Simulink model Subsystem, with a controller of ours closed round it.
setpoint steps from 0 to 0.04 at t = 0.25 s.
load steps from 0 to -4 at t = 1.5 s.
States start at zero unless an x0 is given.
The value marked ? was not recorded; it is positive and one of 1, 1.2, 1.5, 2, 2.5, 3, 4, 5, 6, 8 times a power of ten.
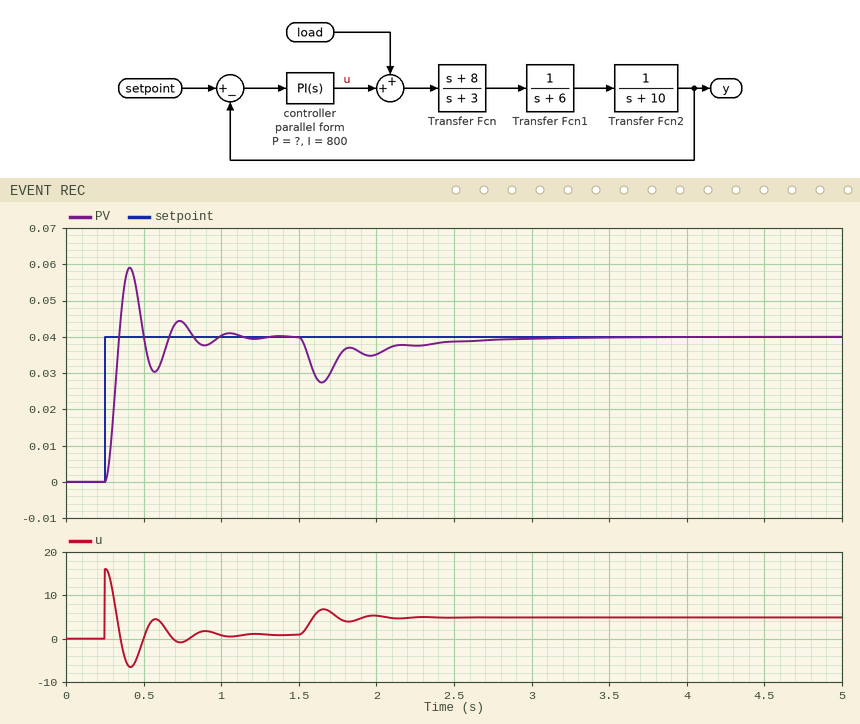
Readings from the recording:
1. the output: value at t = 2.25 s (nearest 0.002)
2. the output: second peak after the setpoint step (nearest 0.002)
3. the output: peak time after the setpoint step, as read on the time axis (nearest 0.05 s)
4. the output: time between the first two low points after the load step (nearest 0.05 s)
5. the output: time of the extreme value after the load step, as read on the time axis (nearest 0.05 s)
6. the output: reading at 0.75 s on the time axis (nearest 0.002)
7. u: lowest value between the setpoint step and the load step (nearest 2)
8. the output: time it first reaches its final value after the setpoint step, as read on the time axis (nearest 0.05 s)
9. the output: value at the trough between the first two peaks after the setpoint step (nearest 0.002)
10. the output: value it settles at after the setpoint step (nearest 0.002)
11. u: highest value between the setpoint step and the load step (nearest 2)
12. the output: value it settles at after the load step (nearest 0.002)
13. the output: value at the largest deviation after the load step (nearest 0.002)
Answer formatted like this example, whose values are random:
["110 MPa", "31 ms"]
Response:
["0.038", "0.044", "0.40 s", "0.30 s", "1.65 s", "0.044", "-6", "0.35 s", "0.030", "0.040", "16", "0.040", "0.028"]
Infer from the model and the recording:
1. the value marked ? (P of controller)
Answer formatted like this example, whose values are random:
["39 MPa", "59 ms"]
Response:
["400"]
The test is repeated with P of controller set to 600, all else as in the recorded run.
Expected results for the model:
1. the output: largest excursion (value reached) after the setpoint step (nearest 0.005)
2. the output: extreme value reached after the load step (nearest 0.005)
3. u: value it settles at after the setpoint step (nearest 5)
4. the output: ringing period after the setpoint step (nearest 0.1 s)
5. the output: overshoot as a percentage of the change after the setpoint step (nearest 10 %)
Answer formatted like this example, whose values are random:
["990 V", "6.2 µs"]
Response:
["0.060", "0.030", "0", "0.3 s", "50 %"]
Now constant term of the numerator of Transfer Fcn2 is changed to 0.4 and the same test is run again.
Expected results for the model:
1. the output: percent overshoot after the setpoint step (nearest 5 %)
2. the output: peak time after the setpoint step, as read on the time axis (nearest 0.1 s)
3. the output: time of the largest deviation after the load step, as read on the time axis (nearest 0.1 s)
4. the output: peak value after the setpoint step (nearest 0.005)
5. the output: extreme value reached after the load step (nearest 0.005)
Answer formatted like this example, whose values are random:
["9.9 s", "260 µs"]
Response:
["30 %", "0.5 s", "1.7 s", "0.050", "0.030"]
